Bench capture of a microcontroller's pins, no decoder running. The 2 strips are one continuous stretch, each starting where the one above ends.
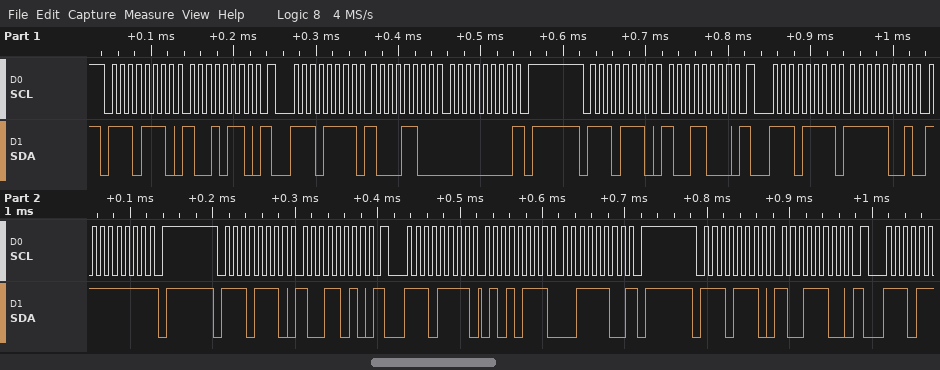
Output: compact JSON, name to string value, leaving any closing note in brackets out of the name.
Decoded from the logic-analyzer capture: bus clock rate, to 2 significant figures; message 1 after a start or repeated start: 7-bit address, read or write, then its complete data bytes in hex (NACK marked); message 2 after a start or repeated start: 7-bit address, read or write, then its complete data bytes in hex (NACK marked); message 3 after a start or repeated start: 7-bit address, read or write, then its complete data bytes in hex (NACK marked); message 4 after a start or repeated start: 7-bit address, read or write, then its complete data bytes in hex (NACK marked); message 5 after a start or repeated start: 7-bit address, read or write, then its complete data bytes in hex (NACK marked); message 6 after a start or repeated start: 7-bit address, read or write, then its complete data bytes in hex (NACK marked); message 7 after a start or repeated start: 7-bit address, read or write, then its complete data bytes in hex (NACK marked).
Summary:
{"bus clock rate, to 2 significant figures": "100 kHz", "message 1 after a start or repeated start: 7-bit address, read or write, then its complete data bytes in hex": "0x77 write: 96", "message 2 after a start or repeated start: 7-bit address, read or write, then its complete data bytes in hex": "0x77 read: 8C 00 NACK", "message 3 after a start or repeated start: 7-bit address, read or write, then its complete data bytes in hex": "0x77 write: 98", "message 4 after a start or repeated start: 7-bit address, read or write, then its complete data bytes in hex": "0x77 read: F9 FF NACK", "message 5 after a start or repeated start: 7-bit address, read or write, then its complete data bytes in hex": "0x77 write: 9A", "message 6 after a start or repeated start: 7-bit address, read or write, then its complete data bytes in hex": "0x77 read: 57 3C NACK", "message 7 after a start or repeated start: 7-bit address, read or write, then its complete data bytes in hex": "0x77 write: 9C"}
